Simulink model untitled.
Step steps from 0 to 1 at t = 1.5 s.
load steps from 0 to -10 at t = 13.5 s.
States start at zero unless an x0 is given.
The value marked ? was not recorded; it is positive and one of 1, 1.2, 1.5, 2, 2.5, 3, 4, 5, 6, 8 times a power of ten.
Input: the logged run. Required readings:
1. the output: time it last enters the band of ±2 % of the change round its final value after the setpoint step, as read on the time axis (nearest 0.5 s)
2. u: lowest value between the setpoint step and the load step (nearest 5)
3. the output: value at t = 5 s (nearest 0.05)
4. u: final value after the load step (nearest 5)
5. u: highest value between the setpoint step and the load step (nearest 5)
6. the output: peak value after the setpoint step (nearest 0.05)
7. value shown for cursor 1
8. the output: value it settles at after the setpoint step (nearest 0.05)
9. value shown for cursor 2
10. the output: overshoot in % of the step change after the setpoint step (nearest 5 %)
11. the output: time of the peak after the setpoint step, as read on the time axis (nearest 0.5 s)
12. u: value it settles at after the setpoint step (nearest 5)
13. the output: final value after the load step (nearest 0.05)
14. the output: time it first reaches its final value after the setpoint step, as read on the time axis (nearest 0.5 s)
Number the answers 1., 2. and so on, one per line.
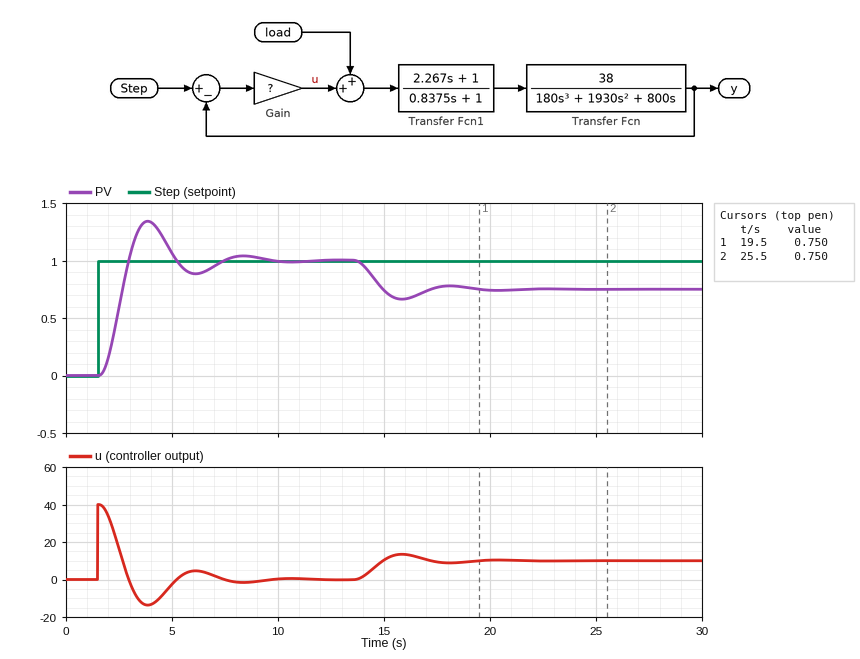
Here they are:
1. 9.0 s
2. -15
3. 1.05
4. 10
5. 40
6. 1.35
7. 0.750
8. 1.00
9. 0.750
10. 35 %
11. 4.0 s
12. 0
13. 0.75
14. 3.0 s
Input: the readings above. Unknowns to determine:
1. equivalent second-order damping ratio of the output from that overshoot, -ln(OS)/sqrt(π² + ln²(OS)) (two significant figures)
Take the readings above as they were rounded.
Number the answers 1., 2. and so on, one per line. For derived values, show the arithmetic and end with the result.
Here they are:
1. ln(0.35) = -1.050; 1.050 / sqrt(9.870 + 1.102) = 0.32
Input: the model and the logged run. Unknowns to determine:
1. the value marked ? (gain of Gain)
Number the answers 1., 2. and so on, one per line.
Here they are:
1. 40
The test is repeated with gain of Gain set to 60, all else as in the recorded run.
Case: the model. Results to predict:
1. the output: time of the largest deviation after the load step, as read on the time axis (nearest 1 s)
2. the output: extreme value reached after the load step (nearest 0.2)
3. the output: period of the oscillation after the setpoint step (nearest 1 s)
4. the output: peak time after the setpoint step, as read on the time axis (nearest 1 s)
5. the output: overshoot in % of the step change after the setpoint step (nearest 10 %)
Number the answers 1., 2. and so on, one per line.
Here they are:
1. 15 s
2. 0.8
3. 4 s
4. 3 s
5. 50 %
